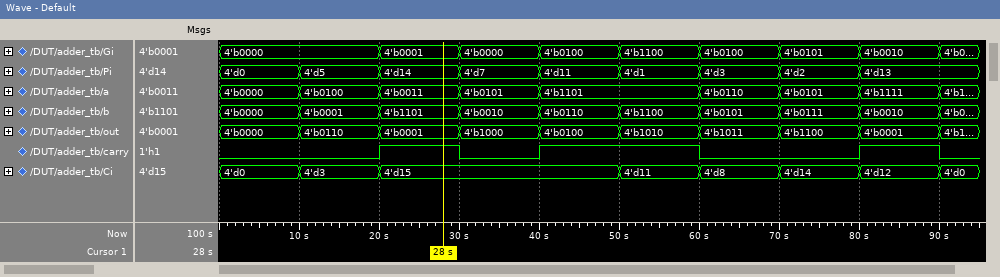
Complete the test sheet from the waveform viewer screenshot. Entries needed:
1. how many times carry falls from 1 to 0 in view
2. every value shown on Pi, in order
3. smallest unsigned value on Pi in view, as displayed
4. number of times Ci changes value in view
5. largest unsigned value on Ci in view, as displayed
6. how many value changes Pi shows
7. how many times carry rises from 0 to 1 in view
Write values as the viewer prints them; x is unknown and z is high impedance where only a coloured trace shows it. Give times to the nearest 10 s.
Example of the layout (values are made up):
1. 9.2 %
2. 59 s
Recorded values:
1. 3
2. 4'd0, 4'd5, 4'd14, 4'd7, 4'd11, 4'd1, 4'd3, 4'd2, 4'd13
3. 4'd0
4. 7
5. 4'd15
6. 8
7. 3
